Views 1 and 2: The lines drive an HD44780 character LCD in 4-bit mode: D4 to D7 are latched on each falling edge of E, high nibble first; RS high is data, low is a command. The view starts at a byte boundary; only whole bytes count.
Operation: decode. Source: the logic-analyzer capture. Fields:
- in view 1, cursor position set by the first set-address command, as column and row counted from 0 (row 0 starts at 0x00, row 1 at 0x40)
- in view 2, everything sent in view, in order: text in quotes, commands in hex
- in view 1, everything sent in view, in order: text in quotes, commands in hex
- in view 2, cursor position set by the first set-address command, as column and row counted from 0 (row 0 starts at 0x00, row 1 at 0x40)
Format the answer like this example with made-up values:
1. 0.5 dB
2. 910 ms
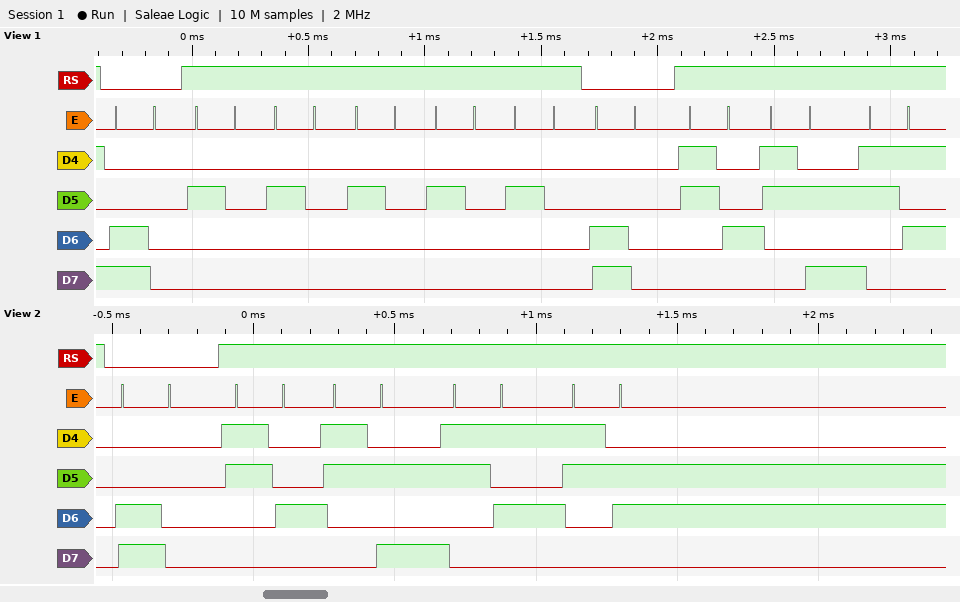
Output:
1. column 0, row 1
2. 0xC0 "4:56"
3. 0xC0 "     " 0xC0 "4:5"
4. column 0, row 1
